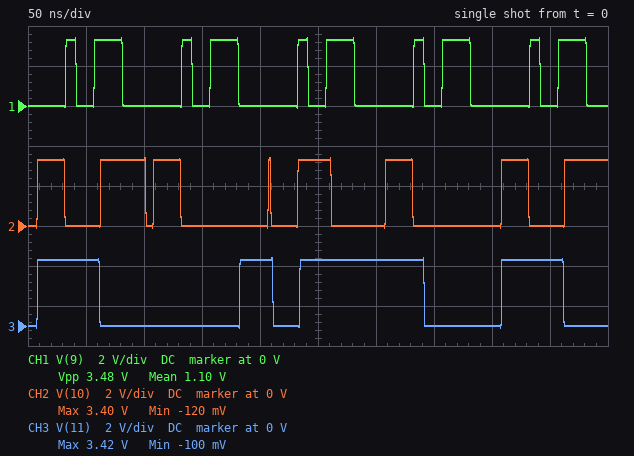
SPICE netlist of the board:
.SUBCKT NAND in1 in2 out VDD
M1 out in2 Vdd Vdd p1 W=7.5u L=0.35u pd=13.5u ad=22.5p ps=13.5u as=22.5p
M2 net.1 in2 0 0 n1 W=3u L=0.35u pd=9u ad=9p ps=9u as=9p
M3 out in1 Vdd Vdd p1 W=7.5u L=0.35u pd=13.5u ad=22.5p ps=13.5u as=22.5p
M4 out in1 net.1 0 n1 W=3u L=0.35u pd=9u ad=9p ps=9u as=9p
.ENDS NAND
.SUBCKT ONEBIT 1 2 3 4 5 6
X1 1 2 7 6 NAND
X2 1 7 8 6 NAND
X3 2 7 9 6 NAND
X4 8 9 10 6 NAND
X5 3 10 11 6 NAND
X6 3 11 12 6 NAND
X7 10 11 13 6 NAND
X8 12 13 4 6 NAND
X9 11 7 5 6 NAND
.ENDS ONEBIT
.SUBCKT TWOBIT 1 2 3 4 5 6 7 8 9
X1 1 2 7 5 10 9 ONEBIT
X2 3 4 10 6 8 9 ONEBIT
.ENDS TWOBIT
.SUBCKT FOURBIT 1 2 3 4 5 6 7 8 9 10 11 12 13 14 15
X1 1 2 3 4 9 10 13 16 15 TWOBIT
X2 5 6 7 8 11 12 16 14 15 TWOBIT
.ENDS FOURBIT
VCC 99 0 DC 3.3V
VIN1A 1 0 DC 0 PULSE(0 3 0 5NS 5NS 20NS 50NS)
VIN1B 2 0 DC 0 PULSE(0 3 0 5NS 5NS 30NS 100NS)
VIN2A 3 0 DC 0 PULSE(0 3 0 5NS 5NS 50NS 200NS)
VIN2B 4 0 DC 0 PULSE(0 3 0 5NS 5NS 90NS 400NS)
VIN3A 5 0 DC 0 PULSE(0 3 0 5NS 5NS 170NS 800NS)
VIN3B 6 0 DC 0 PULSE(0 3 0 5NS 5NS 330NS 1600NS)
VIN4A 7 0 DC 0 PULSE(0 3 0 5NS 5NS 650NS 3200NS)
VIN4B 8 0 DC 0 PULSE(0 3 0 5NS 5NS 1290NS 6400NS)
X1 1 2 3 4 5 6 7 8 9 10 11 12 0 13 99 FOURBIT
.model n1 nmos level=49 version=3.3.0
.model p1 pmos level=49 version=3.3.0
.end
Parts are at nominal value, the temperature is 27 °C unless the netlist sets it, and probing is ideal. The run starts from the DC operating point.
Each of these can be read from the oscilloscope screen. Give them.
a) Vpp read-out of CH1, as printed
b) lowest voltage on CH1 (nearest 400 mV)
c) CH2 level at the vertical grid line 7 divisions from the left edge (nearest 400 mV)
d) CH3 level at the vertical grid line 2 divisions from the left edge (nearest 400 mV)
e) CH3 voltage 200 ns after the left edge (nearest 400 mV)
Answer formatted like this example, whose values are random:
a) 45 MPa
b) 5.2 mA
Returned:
a) 3.48 V
b) 0 V
c) 0 V
d) 0 V
e) 3.2 V
